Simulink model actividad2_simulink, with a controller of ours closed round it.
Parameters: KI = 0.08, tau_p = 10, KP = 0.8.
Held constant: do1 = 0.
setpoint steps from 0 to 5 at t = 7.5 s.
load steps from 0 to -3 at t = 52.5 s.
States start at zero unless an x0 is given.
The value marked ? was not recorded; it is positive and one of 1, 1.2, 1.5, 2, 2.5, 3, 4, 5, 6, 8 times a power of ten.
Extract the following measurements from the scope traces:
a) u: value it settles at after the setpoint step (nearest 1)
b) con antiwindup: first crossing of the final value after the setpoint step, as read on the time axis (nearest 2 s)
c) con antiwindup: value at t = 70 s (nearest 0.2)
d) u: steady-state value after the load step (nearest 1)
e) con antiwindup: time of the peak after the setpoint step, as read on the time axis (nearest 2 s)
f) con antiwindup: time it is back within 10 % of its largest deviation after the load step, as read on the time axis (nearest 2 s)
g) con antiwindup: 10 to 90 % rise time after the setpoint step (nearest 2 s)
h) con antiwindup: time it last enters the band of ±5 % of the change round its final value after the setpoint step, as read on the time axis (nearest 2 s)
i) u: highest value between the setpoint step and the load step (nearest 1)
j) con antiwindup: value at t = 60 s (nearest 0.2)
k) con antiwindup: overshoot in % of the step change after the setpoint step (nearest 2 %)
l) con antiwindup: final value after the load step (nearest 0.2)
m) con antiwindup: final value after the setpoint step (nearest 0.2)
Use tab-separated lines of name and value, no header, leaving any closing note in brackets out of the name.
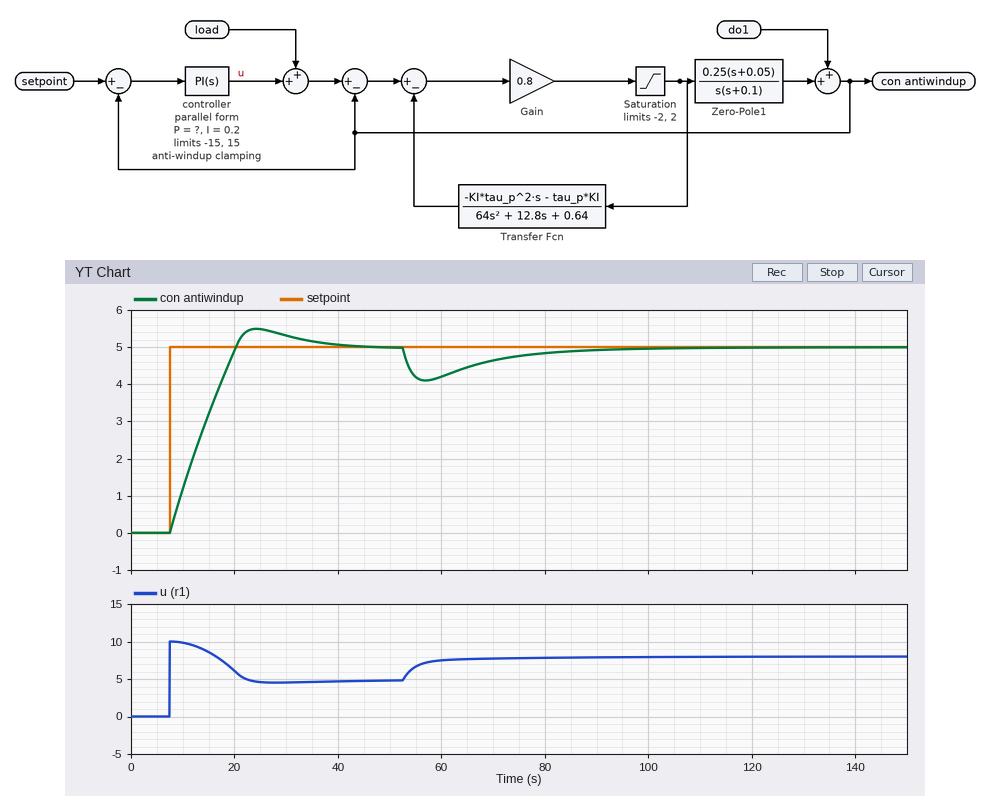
u: value it settles at after the setpoint step	5
con antiwindup: first crossing of the final value after the setpoint step, as read on the time axis	20 s
con antiwindup: value at t = 70 s	4.6
u: steady-state value after the load step	8
con antiwindup: time of the peak after the setpoint step, as read on the time axis	24 s
con antiwindup: time it is back within 10 % of its largest deviation after the load step, as read on the time axis	88 s
con antiwindup: 10 to 90 % rise time after the setpoint step	10 s
con antiwindup: time it last enters the band of ±5 % of the change round its final value after the setpoint step, as read on the time axis	32 s
u: highest value between the setpoint step and the load step	10
con antiwindup: value at t = 60 s	4.2
con antiwindup: overshoot in % of the step change after the setpoint step	10 %
con antiwindup: final value after the load step	5.0
con antiwindup: final value after the setpoint step	5.0
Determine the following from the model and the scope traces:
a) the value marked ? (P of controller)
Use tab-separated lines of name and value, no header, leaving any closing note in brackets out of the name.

the value marked ?	2
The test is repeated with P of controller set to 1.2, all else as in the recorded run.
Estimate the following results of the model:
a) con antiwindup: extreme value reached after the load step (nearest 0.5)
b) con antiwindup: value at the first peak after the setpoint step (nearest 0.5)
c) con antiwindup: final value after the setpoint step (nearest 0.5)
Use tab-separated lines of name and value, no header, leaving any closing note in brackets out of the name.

con antiwindup: extreme value reached after the load step	4.0
con antiwindup: value at the first peak after the setpoint step	5.5
con antiwindup: final value after the setpoint step	5.0
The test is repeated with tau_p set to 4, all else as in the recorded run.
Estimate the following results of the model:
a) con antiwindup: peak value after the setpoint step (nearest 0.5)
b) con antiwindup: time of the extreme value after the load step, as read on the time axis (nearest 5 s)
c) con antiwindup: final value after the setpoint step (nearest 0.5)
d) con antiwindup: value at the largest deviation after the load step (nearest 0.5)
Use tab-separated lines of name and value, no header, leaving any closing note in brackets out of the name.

con antiwindup: peak value after the setpoint step	5.5
con antiwindup: time of the extreme value after the load step, as read on the time axis	55 s
con antiwindup: final value after the setpoint step	5.0
con antiwindup: value at the largest deviation after the load step	4.0
